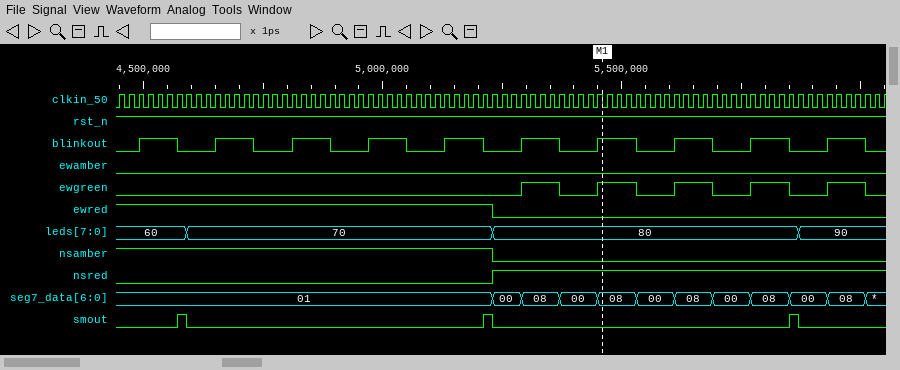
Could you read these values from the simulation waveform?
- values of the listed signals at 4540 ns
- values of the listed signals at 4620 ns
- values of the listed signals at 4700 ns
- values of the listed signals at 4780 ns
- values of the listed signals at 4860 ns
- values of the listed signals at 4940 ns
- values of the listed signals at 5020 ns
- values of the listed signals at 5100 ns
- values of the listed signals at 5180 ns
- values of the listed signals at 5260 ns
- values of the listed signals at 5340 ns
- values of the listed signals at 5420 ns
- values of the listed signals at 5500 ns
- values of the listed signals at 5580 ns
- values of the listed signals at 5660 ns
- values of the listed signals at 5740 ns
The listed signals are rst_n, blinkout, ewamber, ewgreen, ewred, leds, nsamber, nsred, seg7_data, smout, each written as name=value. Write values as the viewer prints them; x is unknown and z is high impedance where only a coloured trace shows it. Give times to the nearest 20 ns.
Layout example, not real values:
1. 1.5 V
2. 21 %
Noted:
1. rst_n=1, blinkout=1, ewamber=0, ewgreen=0, ewred=1, leds=60, nsamber=1, nsred=0, seg7_data=01, smout=0
2. rst_n=1, blinkout=0, ewamber=0, ewgreen=0, ewred=1, leds=70, nsamber=1, nsred=0, seg7_data=01, smout=0
3. rst_n=1, blinkout=1, ewamber=0, ewgreen=0, ewred=1, leds=70, nsamber=1, nsred=0, seg7_data=01, smout=0
4. rst_n=1, blinkout=0, ewamber=0, ewgreen=0, ewred=1, leds=70, nsamber=1, nsred=0, seg7_data=01, smout=0
5. rst_n=1, blinkout=1, ewamber=0, ewgreen=0, ewred=1, leds=70, nsamber=1, nsred=0, seg7_data=01, smout=0
6. rst_n=1, blinkout=0, ewamber=0, ewgreen=0, ewred=1, leds=70, nsamber=1, nsred=0, seg7_data=01, smout=0
7. rst_n=1, blinkout=1, ewamber=0, ewgreen=0, ewred=1, leds=70, nsamber=1, nsred=0, seg7_data=01, smout=0
8. rst_n=1, blinkout=0, ewamber=0, ewgreen=0, ewred=1, leds=70, nsamber=1, nsred=0, seg7_data=01, smout=0
9. rst_n=1, blinkout=1, ewamber=0, ewgreen=0, ewred=1, leds=70, nsamber=1, nsred=0, seg7_data=01, smout=0
10. rst_n=1, blinkout=0, ewamber=0, ewgreen=0, ewred=0, leds=80, nsamber=0, nsred=1, seg7_data=00, smout=0
11. rst_n=1, blinkout=1, ewamber=0, ewgreen=1, ewred=0, leds=80, nsamber=0, nsred=1, seg7_data=08, smout=0
12. rst_n=1, blinkout=0, ewamber=0, ewgreen=0, ewred=0, leds=80, nsamber=0, nsred=1, seg7_data=00, smout=0
13. rst_n=1, blinkout=1, ewamber=0, ewgreen=1, ewred=0, leds=80, nsamber=0, nsred=1, seg7_data=08, smout=0
14. rst_n=1, blinkout=0, ewamber=0, ewgreen=0, ewred=0, leds=80, nsamber=0, nsred=1, seg7_data=00, smout=0
15. rst_n=1, blinkout=1, ewamber=0, ewgreen=1, ewred=0, leds=80, nsamber=0, nsred=1, seg7_data=08, smout=0
16. rst_n=1, blinkout=0, ewamber=0, ewgreen=0, ewred=0, leds=80, nsamber=0, nsred=1, seg7_data=00, smout=0
